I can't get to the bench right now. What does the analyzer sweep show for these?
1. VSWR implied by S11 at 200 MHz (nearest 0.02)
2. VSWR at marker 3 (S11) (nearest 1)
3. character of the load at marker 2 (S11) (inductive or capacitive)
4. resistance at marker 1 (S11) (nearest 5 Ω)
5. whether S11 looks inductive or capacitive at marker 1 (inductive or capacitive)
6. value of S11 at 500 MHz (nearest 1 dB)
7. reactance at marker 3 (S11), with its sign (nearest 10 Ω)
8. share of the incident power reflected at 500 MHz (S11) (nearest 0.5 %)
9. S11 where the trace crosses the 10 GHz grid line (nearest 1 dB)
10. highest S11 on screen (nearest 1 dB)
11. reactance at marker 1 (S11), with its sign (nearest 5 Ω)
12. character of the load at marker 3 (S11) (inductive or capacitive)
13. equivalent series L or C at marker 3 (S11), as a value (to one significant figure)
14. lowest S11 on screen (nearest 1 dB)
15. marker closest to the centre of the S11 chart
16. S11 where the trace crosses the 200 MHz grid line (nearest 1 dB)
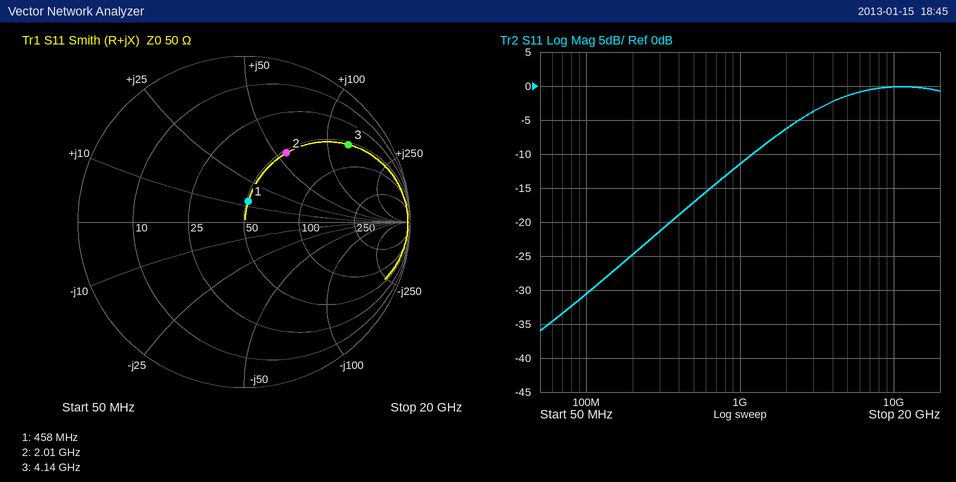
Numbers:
1.12
8
inductive
50 Ω
inductive
-17 dB
+130 Ω
2.0 %
0 dB
0 dB
+15 Ω
inductive
5 nH
-36 dB
marker 1
-25 dB
